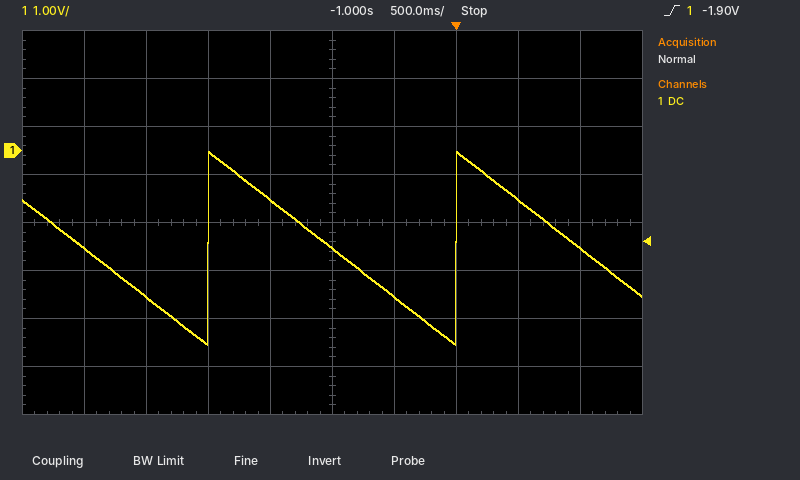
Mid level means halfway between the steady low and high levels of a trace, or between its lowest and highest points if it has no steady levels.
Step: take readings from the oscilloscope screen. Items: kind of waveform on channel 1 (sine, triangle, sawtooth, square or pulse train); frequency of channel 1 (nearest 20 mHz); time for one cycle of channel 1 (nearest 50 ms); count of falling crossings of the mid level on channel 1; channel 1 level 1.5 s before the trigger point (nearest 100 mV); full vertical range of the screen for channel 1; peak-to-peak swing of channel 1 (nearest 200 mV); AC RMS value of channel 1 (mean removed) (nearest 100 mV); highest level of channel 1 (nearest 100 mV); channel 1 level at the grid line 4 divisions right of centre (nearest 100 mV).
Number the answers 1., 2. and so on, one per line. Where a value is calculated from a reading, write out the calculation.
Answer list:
1. sawtooth
2. 1 / 2.00 s ≈ 500 mHz
3. 2.00 s
4. 3
5. -1.0 V
6. 8 V
7. 4.0 V
8. 4.0 V / (2√3) ≈ 1.2 V
9. 0.0 V
10. -2.0 V
